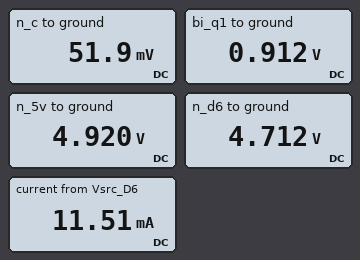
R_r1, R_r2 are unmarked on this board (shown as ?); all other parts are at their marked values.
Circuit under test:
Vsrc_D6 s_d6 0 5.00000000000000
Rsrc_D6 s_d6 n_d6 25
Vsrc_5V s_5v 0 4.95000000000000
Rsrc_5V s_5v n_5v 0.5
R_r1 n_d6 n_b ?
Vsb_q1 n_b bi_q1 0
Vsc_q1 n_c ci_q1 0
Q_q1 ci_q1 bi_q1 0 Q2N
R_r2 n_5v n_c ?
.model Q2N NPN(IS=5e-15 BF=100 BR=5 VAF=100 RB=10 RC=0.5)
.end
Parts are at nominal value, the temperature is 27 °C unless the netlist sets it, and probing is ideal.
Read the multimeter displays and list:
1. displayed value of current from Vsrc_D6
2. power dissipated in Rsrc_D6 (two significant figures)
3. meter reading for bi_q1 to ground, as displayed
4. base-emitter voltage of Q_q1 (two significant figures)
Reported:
11.51 mA
3.3 mW
0.912 V
910 mV
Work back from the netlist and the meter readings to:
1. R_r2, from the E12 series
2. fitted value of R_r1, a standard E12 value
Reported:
82 Ω
330 Ω
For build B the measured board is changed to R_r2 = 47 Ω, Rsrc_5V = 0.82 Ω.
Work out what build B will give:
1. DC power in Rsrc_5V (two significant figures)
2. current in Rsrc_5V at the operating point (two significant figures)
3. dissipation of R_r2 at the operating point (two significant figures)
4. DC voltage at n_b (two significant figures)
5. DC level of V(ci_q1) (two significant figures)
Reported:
8.5 mW
100 mA
490 mW
920 mV
82 mV
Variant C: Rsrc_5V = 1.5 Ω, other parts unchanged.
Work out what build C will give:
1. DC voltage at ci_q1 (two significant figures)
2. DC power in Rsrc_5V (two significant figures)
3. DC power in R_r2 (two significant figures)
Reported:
51 mV
5.2 mW
280 mW
